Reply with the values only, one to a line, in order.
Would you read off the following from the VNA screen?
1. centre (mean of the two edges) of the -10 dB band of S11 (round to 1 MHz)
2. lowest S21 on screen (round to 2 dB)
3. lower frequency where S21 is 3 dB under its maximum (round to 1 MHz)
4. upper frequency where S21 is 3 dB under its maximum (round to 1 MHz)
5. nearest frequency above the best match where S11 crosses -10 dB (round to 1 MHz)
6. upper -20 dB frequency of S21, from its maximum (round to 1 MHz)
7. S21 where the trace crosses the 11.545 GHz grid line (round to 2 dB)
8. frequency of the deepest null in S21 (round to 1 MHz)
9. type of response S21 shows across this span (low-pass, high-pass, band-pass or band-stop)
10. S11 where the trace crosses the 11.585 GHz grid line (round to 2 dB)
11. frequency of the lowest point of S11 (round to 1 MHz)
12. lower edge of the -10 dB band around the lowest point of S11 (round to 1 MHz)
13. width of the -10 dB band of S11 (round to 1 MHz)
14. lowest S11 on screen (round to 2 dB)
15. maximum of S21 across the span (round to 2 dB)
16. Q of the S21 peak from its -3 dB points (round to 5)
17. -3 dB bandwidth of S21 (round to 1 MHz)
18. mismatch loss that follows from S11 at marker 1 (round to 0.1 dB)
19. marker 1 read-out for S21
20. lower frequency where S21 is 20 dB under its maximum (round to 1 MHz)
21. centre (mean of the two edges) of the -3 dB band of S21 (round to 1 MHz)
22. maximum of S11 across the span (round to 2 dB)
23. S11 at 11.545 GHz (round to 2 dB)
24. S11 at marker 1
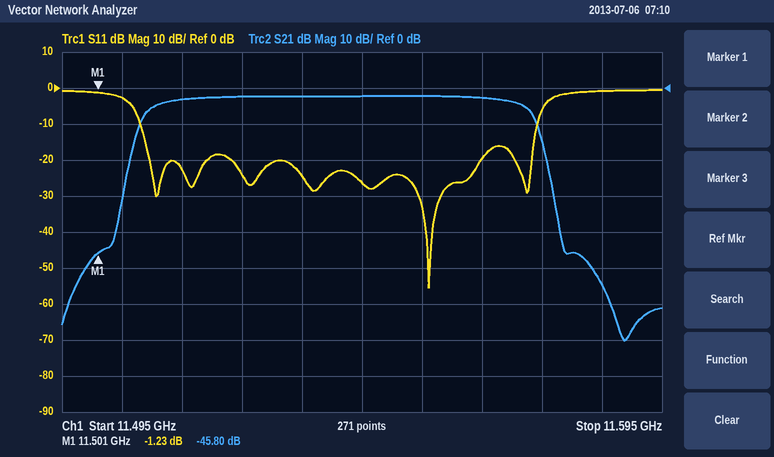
11.541 GHz
-70 dB
11.510 GHz
11.572 GHz
11.574 GHz
11.576 GHz
-2 dB
11.589 GHz
band-pass
0 dB
11.556 GHz
11.508 GHz
66 MHz
-56 dB
-2 dB
185
62 MHz
6.1 dB
-45.80 dB
11.506 GHz
11.541 GHz
0 dB
-26 dB
-1.23 dB
